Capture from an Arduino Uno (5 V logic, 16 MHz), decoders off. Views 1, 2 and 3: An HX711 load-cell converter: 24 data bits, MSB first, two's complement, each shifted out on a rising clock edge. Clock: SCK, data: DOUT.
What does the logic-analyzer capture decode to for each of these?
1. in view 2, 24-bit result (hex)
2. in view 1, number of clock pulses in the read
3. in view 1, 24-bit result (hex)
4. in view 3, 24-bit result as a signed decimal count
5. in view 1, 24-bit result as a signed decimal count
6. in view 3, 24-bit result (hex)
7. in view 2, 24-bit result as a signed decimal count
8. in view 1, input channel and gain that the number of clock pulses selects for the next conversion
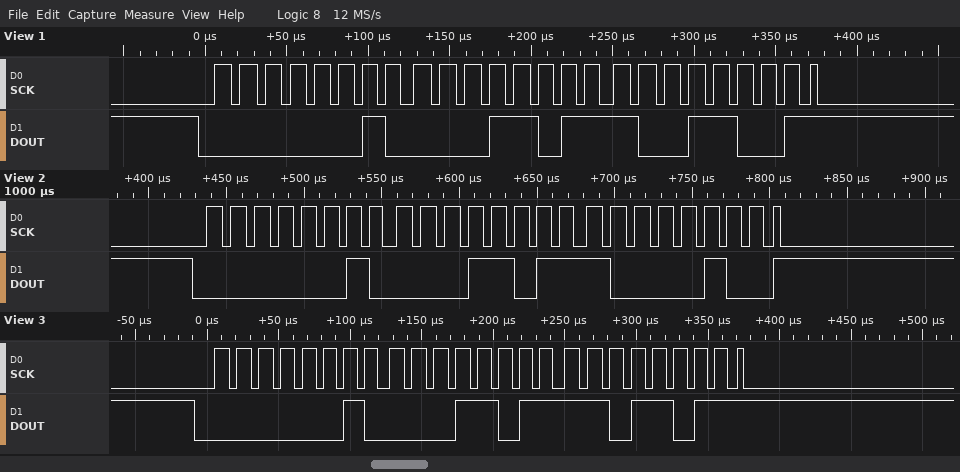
0x021B84
25
0x021B99
138203
138137
0x021BDB
138116
channel A, gain 128
